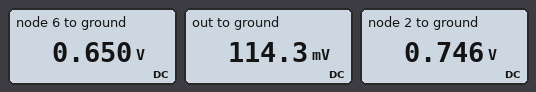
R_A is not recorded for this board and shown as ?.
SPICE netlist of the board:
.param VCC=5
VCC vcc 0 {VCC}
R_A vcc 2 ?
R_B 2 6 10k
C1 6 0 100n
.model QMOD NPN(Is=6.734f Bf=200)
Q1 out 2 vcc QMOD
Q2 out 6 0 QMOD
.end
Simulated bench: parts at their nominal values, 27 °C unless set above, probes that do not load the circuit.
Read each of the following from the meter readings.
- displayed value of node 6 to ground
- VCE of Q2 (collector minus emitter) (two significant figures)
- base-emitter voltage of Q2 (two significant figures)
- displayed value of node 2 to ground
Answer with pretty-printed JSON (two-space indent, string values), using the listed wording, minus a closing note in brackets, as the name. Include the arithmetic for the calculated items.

{
  "displayed value of node 6 to ground": "0.650 V",
  "VCE of Q2 (collector minus emitter)": "114.3 mV = 110 mV",
  "base-emitter voltage of Q2": "650 mV = 650 mV",
  "displayed value of node 2 to ground": "0.746 V"
}
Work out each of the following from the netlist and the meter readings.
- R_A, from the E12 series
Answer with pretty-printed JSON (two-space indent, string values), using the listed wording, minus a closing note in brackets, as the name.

{
  "R_A, from the E12 series": "15 kΩ"
}
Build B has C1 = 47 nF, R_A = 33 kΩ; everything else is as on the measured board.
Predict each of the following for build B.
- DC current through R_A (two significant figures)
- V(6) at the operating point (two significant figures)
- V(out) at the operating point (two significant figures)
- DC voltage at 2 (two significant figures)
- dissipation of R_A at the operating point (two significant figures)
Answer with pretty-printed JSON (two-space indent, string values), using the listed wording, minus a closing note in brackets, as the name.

{
  "DC current through R_A": "130 µA",
  "V(6) at the operating point": "630 mV",
  "V(out) at the operating point": "96 mV",
  "DC voltage at 2": "710 mV",
  "dissipation of R_A at the operating point": "560 µW"
}
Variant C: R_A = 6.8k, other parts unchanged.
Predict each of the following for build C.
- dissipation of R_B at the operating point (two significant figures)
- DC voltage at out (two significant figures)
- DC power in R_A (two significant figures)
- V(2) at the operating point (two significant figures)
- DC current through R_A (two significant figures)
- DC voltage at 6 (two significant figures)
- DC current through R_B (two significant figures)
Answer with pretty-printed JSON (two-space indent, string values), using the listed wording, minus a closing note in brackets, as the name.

{
  "dissipation of R_B at the operating point": "1.4 µW",
  "DC voltage at out": "140 mV",
  "DC power in R_A": "2.6 mW",
  "V(2) at the operating point": "790 mV",
  "DC current through R_A": "620 µA",
  "DC voltage at 6": "670 mV",
  "DC current through R_B": "12 µA"
}
